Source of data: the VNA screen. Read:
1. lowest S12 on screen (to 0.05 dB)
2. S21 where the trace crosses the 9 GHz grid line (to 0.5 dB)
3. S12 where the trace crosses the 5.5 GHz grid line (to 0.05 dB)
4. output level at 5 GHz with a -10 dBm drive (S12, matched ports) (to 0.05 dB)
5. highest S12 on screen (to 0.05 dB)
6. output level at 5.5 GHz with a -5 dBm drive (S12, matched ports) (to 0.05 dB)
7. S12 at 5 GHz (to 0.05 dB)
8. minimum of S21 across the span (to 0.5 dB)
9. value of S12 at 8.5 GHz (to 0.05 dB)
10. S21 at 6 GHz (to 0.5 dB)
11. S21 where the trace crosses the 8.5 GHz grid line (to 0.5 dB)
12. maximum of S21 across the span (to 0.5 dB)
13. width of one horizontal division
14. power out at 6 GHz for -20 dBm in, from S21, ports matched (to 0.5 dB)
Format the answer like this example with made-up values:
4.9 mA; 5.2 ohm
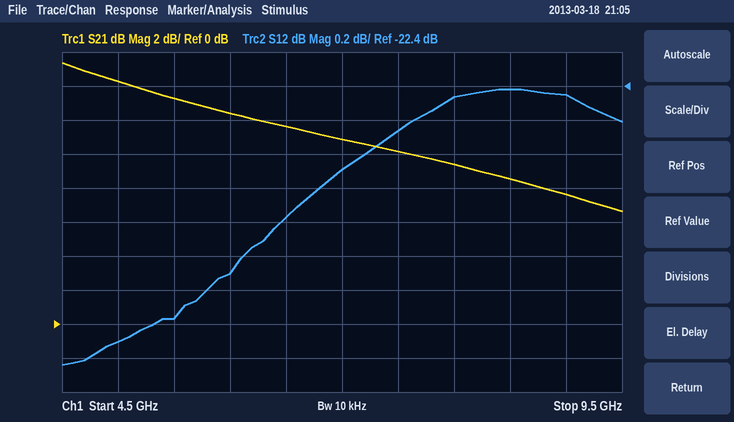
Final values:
-24.05 dB; 7.5 dB; -23.75 dB; -33.90 dBm; -22.40 dB; -28.75 dBm; -23.90 dB; 6.5 dB; -22.40 dB; 12.5 dB; 8.5 dB; 15.5 dB; 500 MHz; -7.5 dBm
